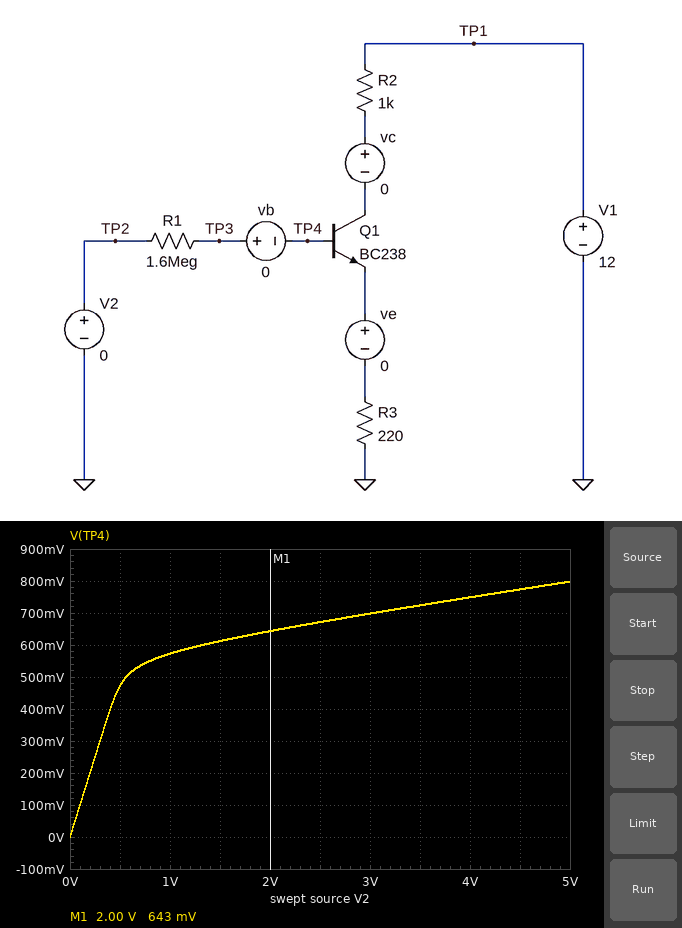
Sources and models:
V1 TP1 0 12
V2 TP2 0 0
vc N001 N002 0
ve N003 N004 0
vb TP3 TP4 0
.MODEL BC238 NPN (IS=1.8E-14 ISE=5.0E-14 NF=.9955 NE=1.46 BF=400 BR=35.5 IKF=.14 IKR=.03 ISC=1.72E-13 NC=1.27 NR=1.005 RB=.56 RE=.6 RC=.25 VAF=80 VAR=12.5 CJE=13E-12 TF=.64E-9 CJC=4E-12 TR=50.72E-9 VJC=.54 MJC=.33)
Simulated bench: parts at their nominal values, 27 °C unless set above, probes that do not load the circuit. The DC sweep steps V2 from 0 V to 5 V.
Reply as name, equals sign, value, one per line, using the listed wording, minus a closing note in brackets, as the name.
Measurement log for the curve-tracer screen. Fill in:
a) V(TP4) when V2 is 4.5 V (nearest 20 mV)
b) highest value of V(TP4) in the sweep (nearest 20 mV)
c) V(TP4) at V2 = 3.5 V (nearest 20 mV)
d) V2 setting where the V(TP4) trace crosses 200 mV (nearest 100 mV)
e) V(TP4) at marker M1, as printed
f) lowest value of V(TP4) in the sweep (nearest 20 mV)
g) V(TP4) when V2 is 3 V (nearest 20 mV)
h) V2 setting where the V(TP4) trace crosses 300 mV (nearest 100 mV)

V(TP4) when V2 is 4.5 V = 780 mV
highest value of V(TP4) in the sweep = 800 mV
V(TP4) at V2 = 3.5 V = 720 mV
V2 setting where the V(TP4) trace crosses 200 mV = 200 mV
V(TP4) at marker M1, as printed = 643 mV
lowest value of V(TP4) in the sweep = 0 V
V(TP4) when V2 is 3 V = 700 mV
V2 setting where the V(TP4) trace crosses 300 mV = 300 mV
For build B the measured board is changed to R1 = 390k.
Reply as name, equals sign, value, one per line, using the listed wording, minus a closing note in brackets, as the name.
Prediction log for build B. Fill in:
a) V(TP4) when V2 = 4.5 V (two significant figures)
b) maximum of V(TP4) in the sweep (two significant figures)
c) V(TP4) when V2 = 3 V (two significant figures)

V(TP4) when V2 = 4.5 V = 1.2 V
maximum of V(TP4) in the sweep = 1.3 V
V(TP4) when V2 = 3 V = 1.0 V
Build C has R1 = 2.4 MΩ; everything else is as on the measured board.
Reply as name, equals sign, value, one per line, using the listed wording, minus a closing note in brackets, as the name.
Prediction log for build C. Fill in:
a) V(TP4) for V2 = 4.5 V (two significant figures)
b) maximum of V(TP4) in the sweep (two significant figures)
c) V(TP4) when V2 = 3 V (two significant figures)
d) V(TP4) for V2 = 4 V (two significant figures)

V(TP4) for V2 = 4.5 V = 710 mV
maximum of V(TP4) in the sweep = 730 mV
V(TP4) when V2 = 3 V = 660 mV
V(TP4) for V2 = 4 V = 690 mV
